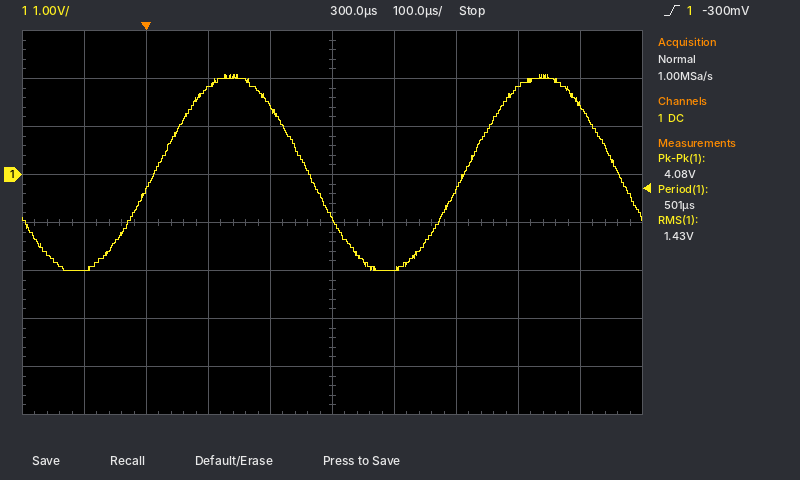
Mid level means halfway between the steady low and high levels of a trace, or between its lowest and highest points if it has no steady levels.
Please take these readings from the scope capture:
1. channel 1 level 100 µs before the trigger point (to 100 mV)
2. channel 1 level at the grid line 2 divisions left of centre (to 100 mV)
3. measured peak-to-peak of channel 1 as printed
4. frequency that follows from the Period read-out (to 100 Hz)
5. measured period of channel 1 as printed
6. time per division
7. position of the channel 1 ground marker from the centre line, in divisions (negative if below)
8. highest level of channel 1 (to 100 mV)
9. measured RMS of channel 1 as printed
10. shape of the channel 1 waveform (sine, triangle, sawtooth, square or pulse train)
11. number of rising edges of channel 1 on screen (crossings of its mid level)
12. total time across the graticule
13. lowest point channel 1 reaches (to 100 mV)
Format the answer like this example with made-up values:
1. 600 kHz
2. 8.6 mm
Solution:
1. -2.0 V
2. 1.8 V
3. 4.08 V
4. 2.0 kHz
5. 501 µs
6. 100 µs
7. +1.0 div
8. 2.1 V
9. 1.43 V
10. sine
11. 2
12. 1 ms
13. -2.0 V
